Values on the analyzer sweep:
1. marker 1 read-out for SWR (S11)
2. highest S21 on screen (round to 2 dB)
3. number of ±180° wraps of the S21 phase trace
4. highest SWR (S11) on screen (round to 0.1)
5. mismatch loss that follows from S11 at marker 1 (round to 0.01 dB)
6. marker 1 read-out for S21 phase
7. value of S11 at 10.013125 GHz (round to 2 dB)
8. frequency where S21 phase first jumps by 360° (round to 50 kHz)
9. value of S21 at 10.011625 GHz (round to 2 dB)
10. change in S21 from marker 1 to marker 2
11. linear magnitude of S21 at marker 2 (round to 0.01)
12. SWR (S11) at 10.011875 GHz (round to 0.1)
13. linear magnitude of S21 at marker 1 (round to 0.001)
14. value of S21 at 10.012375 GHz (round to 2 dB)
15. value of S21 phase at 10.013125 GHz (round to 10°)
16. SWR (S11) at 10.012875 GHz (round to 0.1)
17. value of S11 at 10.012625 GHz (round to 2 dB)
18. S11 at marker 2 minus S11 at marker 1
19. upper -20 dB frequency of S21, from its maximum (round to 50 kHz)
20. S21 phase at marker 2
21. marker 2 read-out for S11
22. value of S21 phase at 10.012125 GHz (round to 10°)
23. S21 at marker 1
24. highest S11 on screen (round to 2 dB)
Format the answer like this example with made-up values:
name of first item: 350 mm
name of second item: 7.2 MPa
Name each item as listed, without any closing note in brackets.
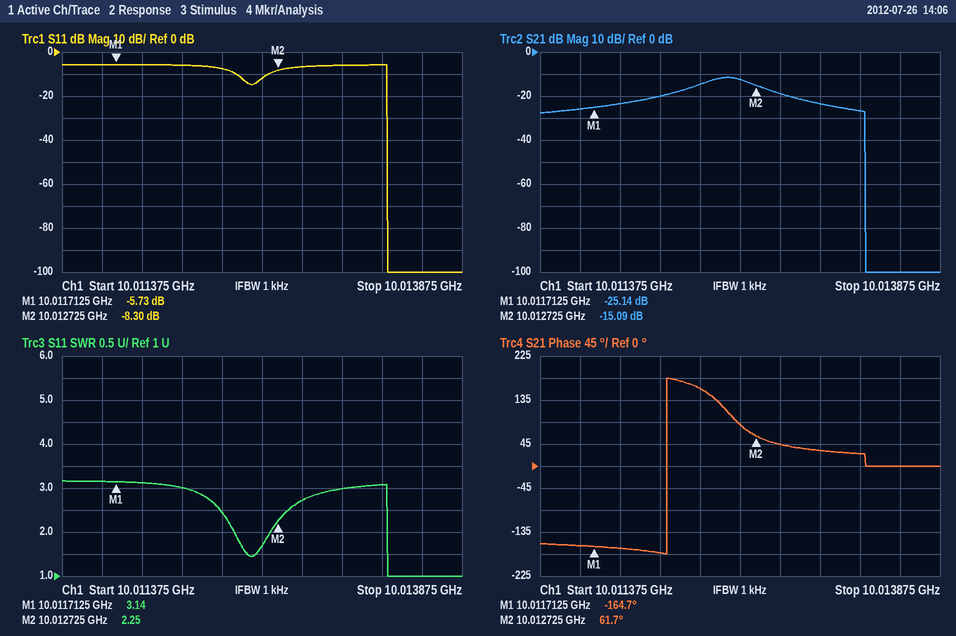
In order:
marker 1 read-out for SWR: 3.14
highest S21 on screen: -12 dB
number of ±180° wraps of the S21 phase trace: 1
highest SWR (S11) on screen: 3.2
mismatch loss that follows from S11 at marker 1: 1.35 dB
marker 1 read-out for S21 phase: -164.7°
value of S11 at 10.013125 GHz: -6 dB
frequency where S21 phase first jumps by 360°: 10.01215 GHz
value of S21 at 10.011625 GHz: -26 dB
change in S21 from marker 1 to marker 2: 10.05 dB
linear magnitude of S21 at marker 2: 0.18
SWR (S11) at 10.011875 GHz: 3.1
linear magnitude of S21 at marker 1: 0.055
value of S21 at 10.012375 GHz: -14 dB
value of S21 phase at 10.013125 GHz: 30°
SWR (S11) at 10.012875 GHz: 2.7
value of S11 at 10.012625 GHz: -12 dB
S11 at marker 2 minus S11 at marker 1: -2.57 dB
upper -20 dB frequency of S21, from its maximum: 10.01340 GHz
S21 phase at marker 2: 61.7°
marker 2 read-out for S11: -8.30 dB
value of S21 phase at 10.012125 GHz: -180°
S21 at marker 1: -25.14 dB
highest S11 on screen: -6 dB
